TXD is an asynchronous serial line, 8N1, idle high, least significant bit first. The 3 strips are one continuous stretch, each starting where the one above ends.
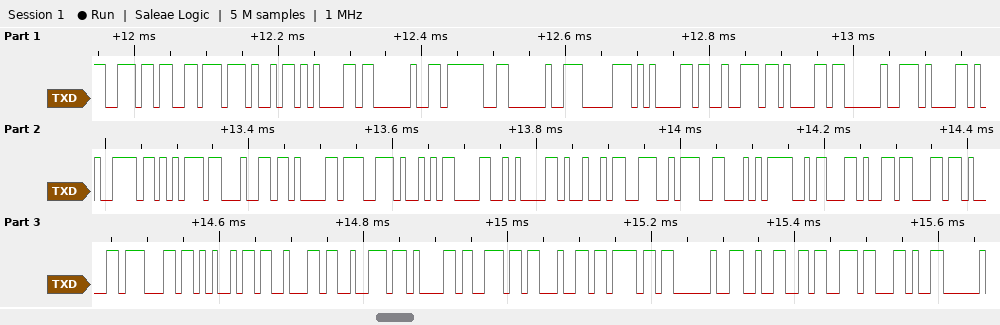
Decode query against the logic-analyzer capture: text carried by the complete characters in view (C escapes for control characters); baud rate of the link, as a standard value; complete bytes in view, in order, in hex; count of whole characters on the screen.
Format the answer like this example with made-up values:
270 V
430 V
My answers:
"nvia ? para ayuda.\r\nINFO,calibrando 2s,"
115200 baud
6E 76 69 61 20 3F 20 70 61 72 61 20 61 79 75 64 61 2E 0D 0A 49 4E 46 4F 2C 63 61 6C 69 62 72 61 6E 64 6F 20 32 73 2C
39
